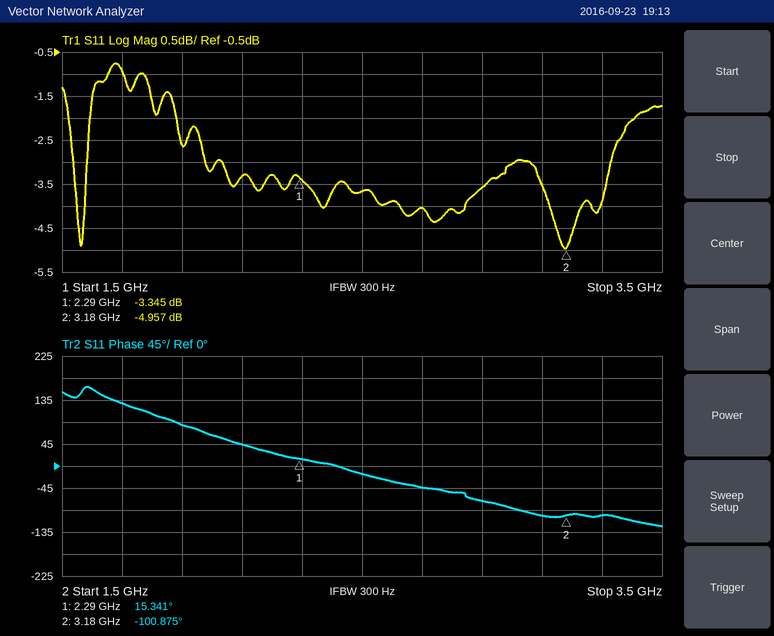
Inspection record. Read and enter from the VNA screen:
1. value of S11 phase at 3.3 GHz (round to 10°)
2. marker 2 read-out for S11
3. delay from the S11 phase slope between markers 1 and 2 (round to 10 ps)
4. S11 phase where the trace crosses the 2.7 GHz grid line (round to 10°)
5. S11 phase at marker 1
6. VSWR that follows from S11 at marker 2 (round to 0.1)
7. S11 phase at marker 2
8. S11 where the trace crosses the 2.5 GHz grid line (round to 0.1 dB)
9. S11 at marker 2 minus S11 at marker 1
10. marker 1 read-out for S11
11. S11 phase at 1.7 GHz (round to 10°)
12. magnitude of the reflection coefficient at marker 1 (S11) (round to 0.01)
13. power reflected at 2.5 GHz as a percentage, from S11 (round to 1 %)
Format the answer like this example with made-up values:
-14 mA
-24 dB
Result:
-100°
-4.957 dB
360 ps
-40°
15.341°
3.6
-100.875°
-3.7 dB
-1.612 dB
-3.345 dB
130°
0.68
43 %
